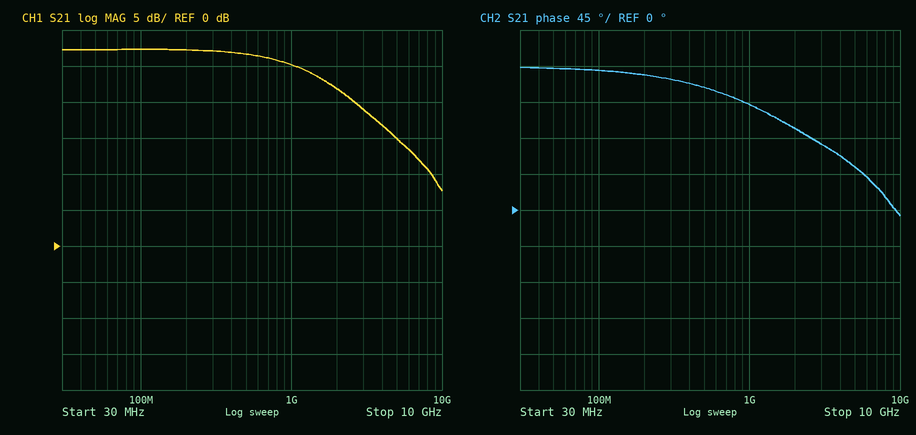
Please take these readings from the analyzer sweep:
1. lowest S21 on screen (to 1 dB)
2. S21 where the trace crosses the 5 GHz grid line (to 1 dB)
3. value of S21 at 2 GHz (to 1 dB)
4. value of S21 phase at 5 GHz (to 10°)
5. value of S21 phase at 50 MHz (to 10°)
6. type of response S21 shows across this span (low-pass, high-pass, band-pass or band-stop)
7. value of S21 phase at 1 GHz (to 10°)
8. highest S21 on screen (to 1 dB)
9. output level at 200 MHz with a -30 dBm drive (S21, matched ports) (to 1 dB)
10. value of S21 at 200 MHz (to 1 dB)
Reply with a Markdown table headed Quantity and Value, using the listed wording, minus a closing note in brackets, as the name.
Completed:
| Quantity | Value |
|---|---|
| lowest S21 on screen | 8 dB |
| S21 where the trace crosses the 5 GHz grid line | 15 dB |
| value of S21 at 2 GHz | 22 dB |
| value of S21 phase at 5 GHz | 50° |
| value of S21 phase at 50 MHz | 180° |
| type of response S21 shows across this span | low-pass |
| value of S21 phase at 1 GHz | 130° |
| highest S21 on screen | 27 dB |
| output level at 200 MHz with a -30 dBm drive (S21, matched ports) | -3 dBm |
| value of S21 at 200 MHz | 27 dB |
